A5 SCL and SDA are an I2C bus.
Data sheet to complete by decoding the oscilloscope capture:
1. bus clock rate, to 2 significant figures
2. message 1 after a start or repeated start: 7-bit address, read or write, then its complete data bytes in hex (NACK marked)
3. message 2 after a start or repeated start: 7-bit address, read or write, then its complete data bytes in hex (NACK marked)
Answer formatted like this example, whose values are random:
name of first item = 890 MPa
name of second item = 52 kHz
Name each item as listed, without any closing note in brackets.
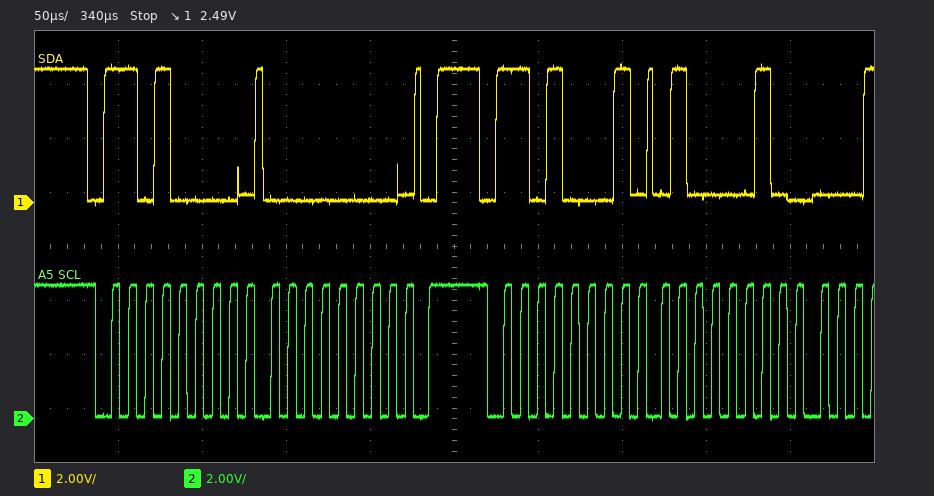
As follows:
bus clock rate, to 2 significant figures = 100 kHz
message 1 after a start or repeated start: 7-bit address, read or write, then its complete data bytes in hex = 0x68 write: 00
message 2 after a start or repeated start: 7-bit address, read or write, then its complete data bytes in hex = 0x68 read: 42
